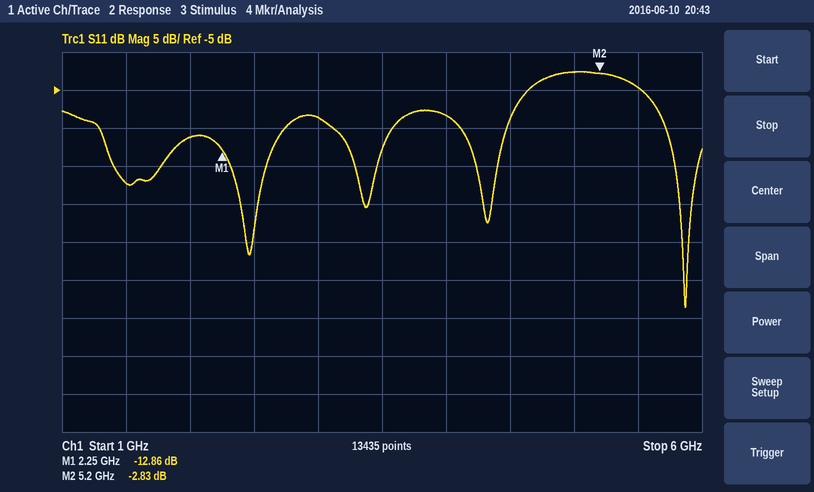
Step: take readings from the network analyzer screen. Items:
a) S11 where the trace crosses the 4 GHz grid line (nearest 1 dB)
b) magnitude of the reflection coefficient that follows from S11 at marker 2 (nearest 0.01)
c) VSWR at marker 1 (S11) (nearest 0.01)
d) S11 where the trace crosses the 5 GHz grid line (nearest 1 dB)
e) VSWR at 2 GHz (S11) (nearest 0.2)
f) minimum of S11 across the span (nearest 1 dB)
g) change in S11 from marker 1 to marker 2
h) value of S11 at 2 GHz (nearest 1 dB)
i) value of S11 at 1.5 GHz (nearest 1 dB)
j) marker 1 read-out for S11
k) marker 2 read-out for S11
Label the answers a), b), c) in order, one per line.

a) -8 dB
b) 0.72
c) 1.59
d) -3 dB
e) 1.8
f) -34 dB
g) 10.03 dB
h) -11 dB
i) -17 dB
j) -12.86 dB
k) -2.83 dB
